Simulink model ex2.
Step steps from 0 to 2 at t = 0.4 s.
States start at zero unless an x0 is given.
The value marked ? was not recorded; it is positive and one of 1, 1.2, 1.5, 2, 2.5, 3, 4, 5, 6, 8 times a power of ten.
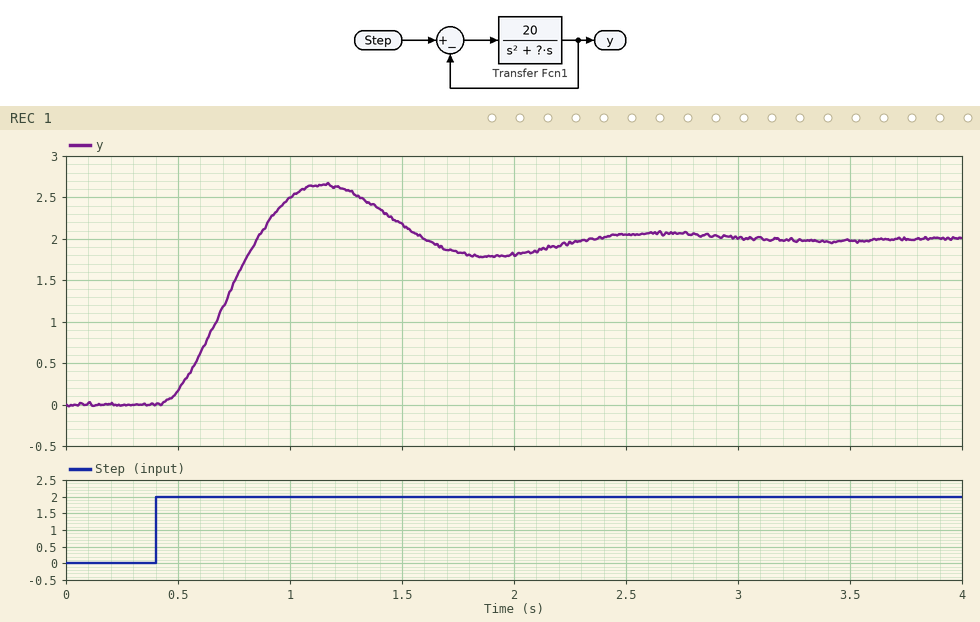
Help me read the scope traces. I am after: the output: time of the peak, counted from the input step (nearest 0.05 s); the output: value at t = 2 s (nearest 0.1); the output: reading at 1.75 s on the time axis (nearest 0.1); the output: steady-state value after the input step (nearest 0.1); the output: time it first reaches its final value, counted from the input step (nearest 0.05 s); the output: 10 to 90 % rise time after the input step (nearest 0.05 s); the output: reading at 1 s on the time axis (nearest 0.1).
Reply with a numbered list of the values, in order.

1. 0.75 s
2. 1.8
3. 1.8
4. 2.0
5. 0.45 s
6. 0.30 s
7. 2.5
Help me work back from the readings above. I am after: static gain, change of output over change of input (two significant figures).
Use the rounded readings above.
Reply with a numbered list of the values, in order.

1. 1.0
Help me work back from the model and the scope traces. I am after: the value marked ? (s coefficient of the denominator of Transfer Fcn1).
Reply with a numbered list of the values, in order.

1. 3
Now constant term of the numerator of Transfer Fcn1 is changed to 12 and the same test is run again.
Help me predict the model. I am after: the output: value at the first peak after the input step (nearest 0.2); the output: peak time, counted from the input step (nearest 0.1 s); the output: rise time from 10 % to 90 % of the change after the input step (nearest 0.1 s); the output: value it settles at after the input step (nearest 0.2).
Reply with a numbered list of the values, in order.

1. 2.4
2. 1.0 s
3. 0.4 s
4. 2.0
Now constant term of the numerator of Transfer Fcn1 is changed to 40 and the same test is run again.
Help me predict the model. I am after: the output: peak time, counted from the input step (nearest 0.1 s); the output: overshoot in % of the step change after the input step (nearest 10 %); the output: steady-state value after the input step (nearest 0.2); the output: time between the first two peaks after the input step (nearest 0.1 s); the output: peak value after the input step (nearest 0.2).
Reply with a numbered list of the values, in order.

1. 0.5 s
2. 50 %
3. 2.0
4. 1.0 s
5. 3.0
